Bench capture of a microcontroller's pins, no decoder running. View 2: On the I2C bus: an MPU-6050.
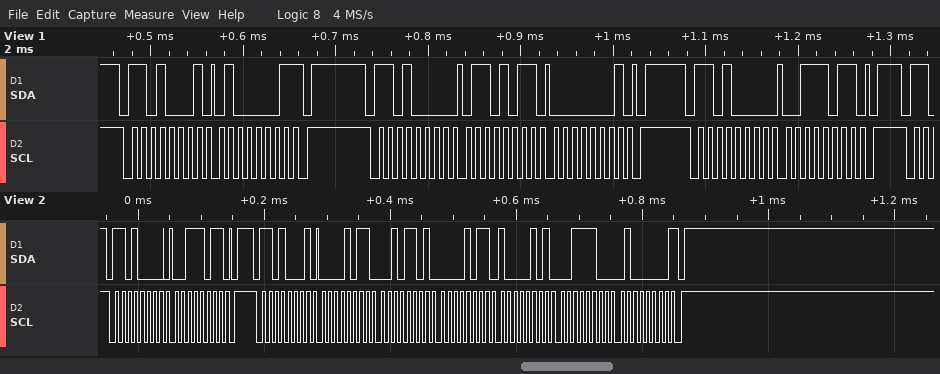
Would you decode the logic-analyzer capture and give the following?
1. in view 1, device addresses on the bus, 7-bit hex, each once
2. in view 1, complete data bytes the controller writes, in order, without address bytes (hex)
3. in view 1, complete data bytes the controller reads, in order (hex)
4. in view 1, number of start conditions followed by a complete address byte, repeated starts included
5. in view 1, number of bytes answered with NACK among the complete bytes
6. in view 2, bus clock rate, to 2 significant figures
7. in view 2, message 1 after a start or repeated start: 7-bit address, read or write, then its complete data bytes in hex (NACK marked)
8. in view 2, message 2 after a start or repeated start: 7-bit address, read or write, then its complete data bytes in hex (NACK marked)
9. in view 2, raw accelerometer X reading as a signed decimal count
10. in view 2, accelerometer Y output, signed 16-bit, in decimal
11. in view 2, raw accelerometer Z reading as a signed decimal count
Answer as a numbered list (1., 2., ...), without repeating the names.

1. 0x68
2. 6B 01 3B
3. 41
4. 3
5. 1
6. 100 kHz
7. 0x68 write: 3B
8. 0x68 read: 0B 2D 0B 85 3C 40 NACK
9. 2861
10. 2949
11. 15424
